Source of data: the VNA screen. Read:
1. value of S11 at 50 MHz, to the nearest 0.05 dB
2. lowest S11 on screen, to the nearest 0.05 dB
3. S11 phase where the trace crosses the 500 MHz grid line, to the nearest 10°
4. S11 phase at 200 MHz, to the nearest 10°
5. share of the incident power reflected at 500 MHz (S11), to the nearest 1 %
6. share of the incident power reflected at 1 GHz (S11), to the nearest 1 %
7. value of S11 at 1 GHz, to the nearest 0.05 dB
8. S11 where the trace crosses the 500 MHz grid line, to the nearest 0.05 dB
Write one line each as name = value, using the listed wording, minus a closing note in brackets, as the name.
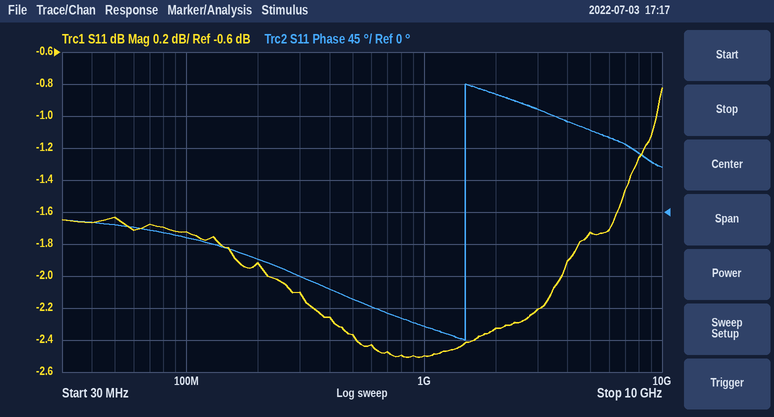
value of S11 at 50 MHz, to the nearest 0.05 dB = -1.65 dB
lowest S11 on screen, to the nearest 0.05 dB = -2.50 dB
S11 phase where the trace crosses the 500 MHz grid line, to the nearest 10° = -120°
S11 phase at 200 MHz, to the nearest 10° = -70°
share of the incident power reflected at 500 MHz (S11), to the nearest 1 % = 58 %
share of the incident power reflected at 1 GHz (S11), to the nearest 1 % = 56 %
value of S11 at 1 GHz, to the nearest 0.05 dB = -2.50 dB
S11 where the trace crosses the 500 MHz grid line, to the nearest 0.05 dB = -2.35 dB
